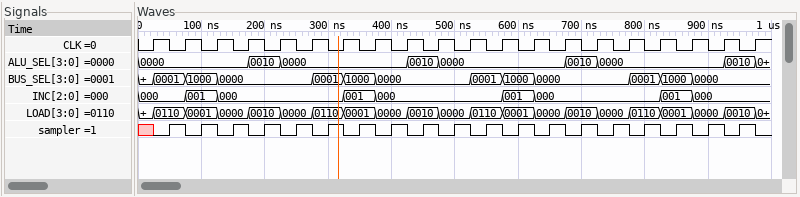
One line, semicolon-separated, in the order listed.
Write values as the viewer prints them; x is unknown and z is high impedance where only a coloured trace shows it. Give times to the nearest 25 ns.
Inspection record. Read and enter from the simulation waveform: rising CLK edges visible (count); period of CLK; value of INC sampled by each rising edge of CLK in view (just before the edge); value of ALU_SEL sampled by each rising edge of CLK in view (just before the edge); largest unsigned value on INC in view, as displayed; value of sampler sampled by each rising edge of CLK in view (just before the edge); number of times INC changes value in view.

20; 50 ns; 000, 000, 001, 000, 000, 000, 000, 001, 000, 000, 000, 000, 001, 000, 000, 000, 000, 001, 000, 000; 0000, 0000, 0000, 0000, 0010, 0000, 0000, 0000, 0000, 0010, 0000, 0000, 0000, 0000, 0010, 0000, 0000, 0000, 0000, 0010; 001; x 1 1 1 1 1 1 1 1 1 1 1 1 1 1 1 1 1 1 1; 8
